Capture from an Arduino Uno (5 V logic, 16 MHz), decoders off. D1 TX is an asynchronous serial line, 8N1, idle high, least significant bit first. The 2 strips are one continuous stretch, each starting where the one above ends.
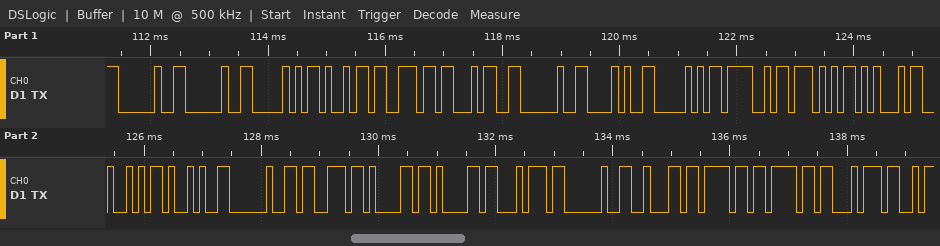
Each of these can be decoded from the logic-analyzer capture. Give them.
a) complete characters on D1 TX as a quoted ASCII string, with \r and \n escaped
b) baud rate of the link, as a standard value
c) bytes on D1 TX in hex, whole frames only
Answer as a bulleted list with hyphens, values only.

- "  Pin4 (POWER) saat boot"
- 9600 baud
- 20 20 50 69 6E 34 20 28 50 4F 57 45 52 29 20 73 61 61 74 20 62 6F 6F 74
